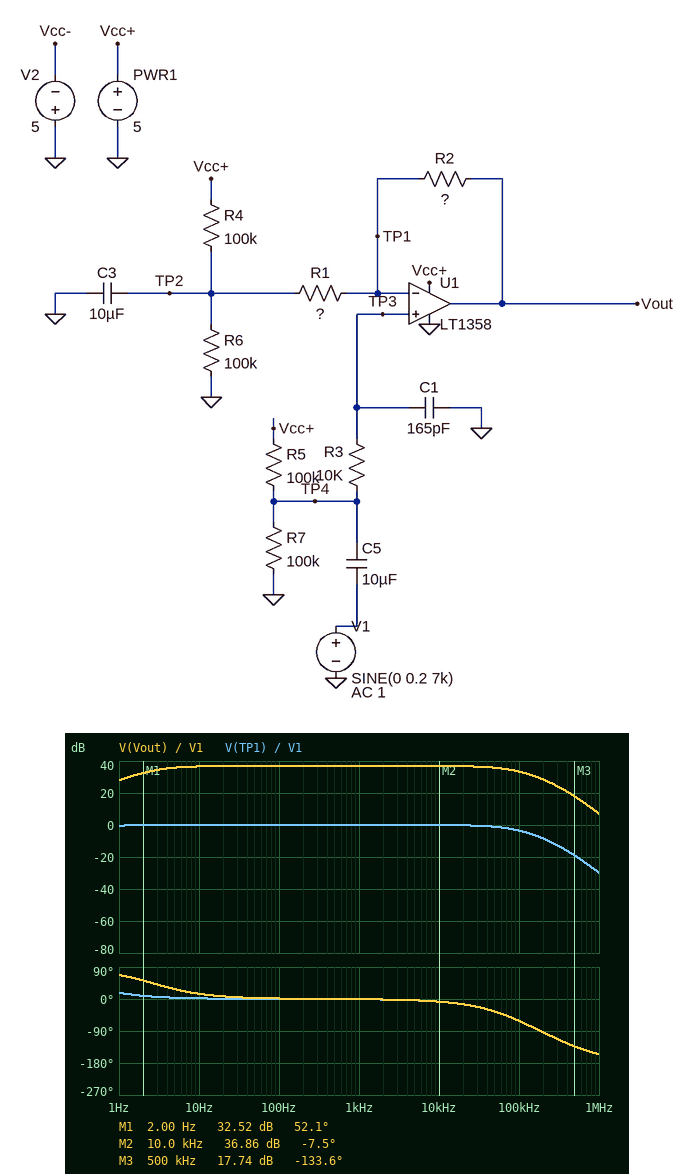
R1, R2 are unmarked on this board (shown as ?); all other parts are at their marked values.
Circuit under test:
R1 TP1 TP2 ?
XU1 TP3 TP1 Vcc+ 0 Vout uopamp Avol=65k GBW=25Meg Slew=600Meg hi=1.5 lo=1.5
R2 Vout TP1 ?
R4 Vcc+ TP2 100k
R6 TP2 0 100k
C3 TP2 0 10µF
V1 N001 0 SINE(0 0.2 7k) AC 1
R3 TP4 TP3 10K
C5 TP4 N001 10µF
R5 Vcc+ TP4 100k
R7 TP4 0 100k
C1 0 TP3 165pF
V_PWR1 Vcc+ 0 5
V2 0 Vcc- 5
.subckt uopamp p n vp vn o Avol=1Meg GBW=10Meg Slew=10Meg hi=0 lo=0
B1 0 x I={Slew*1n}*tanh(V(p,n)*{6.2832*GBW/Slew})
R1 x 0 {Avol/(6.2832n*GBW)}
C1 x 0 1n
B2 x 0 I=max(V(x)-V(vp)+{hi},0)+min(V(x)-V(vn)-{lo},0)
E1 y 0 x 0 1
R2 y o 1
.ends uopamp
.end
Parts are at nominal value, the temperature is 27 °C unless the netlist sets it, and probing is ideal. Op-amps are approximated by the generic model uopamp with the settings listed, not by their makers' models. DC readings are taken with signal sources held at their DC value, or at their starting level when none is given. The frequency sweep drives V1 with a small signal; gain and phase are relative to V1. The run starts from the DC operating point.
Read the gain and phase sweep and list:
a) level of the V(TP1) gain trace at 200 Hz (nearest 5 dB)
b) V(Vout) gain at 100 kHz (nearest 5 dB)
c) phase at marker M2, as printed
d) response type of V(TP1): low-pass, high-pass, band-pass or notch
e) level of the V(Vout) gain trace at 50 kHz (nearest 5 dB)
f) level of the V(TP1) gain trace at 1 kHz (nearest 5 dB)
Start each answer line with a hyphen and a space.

- 0 dB
- 35 dB
- -7.5 deg
- low-pass
- 35 dB
- 0 dB
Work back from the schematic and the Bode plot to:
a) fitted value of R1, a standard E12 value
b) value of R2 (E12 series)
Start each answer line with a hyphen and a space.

- 6.8 kΩ
- 470 kΩ
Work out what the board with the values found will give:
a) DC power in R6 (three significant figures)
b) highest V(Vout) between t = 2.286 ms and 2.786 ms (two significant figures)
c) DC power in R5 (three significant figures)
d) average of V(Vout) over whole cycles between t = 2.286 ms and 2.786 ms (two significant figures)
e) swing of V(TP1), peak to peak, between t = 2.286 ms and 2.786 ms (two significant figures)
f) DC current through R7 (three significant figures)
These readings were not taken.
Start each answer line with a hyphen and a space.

- 62.5 µW
- 3.5 V
- 62.5 µW
- 2.5 V
- 29 mV
- 25.0 µA
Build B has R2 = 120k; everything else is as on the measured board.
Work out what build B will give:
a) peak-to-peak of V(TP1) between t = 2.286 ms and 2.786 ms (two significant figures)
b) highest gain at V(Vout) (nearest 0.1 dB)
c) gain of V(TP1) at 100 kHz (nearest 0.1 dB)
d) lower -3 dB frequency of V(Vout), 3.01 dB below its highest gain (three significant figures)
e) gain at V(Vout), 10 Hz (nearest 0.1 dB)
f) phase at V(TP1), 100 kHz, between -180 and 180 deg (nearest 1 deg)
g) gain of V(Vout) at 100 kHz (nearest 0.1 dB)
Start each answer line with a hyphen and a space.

- 110 mV
- 25.4 dB
- -3.2 dB
- 2.62 Hz
- 25.1 dB
- -50 deg
- 22.2 dB
